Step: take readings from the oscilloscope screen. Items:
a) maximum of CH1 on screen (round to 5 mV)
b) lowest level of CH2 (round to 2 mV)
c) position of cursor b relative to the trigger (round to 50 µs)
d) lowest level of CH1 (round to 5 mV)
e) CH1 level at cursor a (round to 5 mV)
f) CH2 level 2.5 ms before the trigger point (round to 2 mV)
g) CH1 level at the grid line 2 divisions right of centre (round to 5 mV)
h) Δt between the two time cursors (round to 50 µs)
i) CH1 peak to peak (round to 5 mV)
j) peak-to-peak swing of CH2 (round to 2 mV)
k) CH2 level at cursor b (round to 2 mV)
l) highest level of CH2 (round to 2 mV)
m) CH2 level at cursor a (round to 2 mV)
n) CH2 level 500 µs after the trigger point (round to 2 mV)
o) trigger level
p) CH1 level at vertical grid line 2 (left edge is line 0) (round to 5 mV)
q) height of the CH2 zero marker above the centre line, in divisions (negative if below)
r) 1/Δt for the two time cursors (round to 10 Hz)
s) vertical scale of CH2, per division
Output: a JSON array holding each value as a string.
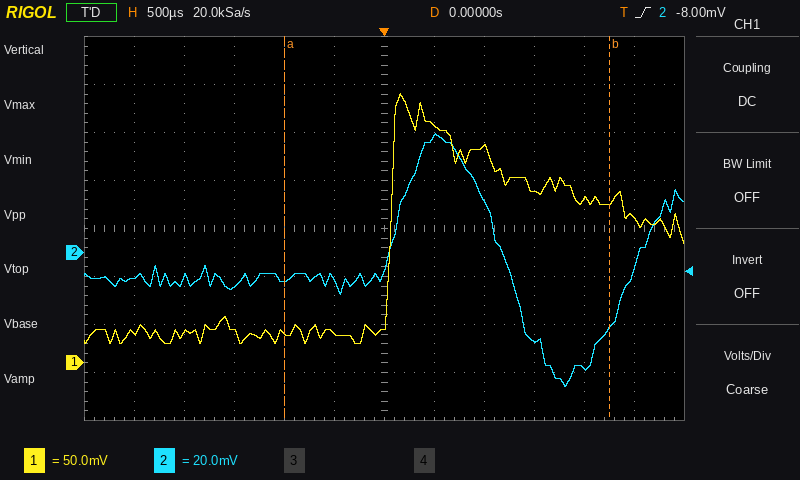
["280 mV", "-56 mV", "+2.25 ms", "20 mV", "30 mV", "-10 mV", "225 mV", "3.25 ms", "260 mV", "106 mV", "-32 mV", "50 mV", "-12 mV", "48 mV", "-8.00 mV", "30 mV", "-0.5 div", "310 Hz", "20 mV"]
